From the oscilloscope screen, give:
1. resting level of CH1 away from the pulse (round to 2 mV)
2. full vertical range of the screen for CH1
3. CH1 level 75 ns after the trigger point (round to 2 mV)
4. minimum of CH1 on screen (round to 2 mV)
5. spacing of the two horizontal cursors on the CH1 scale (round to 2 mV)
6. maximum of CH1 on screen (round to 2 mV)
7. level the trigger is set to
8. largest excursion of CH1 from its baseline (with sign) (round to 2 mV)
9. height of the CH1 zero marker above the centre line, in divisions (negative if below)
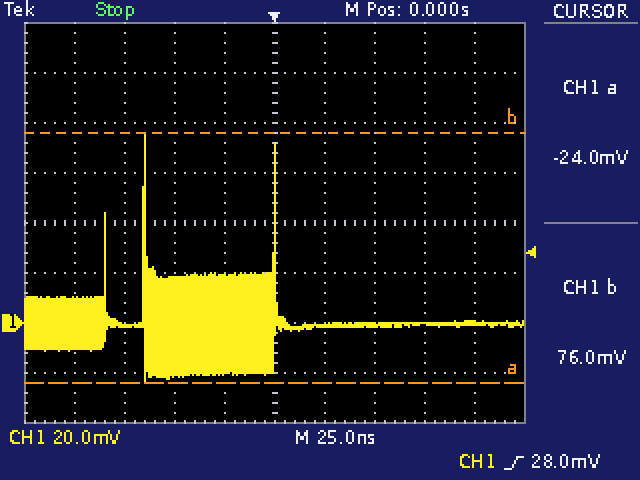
0 mV
160 mV
0 mV
-24 mV
100 mV
76 mV
28.0 mV
+76 mV
-2.0 div
